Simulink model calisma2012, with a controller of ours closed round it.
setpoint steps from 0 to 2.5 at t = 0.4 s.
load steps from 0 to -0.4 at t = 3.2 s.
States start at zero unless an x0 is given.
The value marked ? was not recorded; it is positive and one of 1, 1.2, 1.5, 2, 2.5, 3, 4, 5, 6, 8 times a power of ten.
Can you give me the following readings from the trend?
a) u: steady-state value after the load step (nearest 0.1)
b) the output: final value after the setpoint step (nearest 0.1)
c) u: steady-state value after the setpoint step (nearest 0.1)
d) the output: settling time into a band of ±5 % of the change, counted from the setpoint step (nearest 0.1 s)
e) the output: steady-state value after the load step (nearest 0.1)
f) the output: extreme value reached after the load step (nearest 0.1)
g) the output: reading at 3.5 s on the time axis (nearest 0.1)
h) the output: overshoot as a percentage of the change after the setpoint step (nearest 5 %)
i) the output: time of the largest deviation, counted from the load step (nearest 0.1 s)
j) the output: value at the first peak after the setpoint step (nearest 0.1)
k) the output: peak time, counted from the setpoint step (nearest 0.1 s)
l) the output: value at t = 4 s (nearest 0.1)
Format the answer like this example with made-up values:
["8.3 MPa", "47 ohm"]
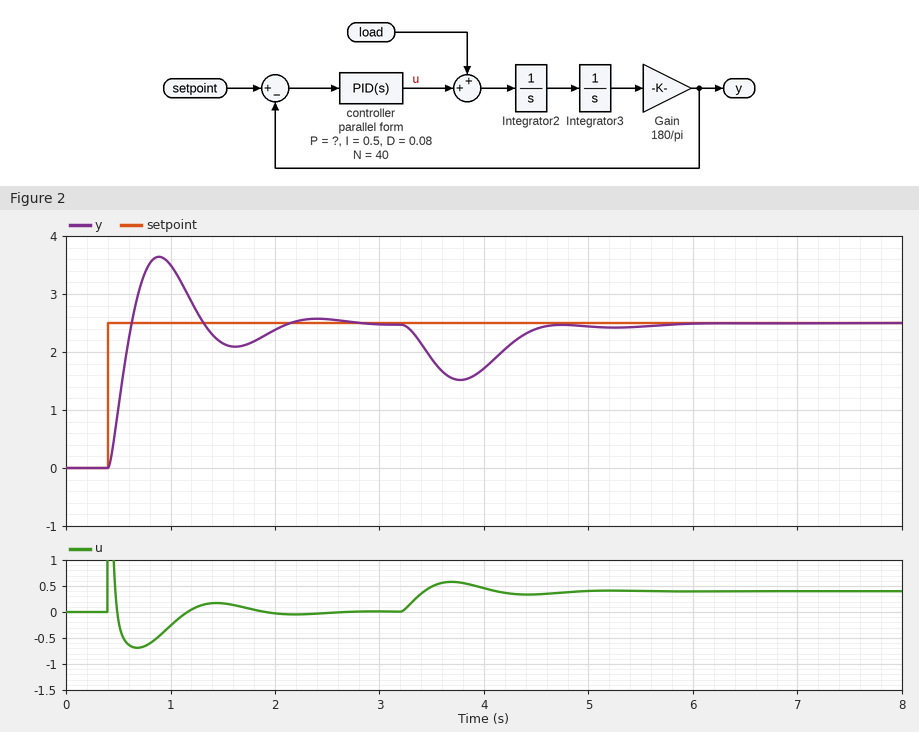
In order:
["0.4", "2.5", "0.0", "1.6 s", "2.5", "1.5", "1.9", "45 %", "0.6 s", "3.6", "0.5 s", "1.7"]
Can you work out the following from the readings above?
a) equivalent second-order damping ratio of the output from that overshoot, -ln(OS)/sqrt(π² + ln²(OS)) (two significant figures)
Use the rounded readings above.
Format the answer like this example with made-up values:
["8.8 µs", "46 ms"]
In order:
["0.25"]
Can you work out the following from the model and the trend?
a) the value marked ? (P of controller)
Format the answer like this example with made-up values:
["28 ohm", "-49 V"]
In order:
["0.4"]
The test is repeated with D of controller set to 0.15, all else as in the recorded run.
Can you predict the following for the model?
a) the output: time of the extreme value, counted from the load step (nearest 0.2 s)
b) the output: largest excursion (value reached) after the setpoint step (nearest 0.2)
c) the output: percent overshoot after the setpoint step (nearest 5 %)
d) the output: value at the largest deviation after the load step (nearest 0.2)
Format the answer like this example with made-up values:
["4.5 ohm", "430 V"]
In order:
["0.6 s", "3.0", "25 %", "1.8"]
